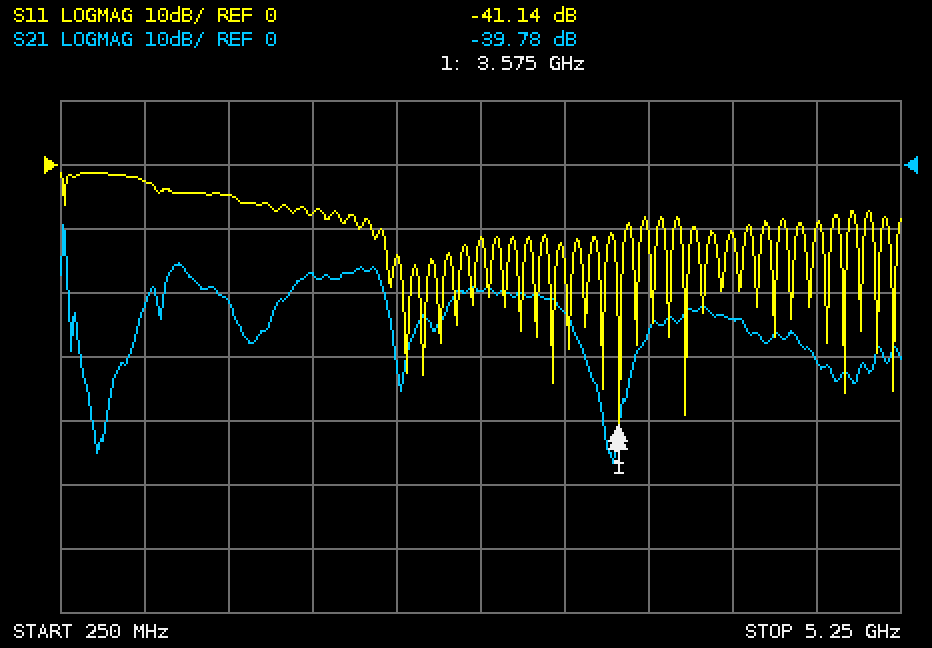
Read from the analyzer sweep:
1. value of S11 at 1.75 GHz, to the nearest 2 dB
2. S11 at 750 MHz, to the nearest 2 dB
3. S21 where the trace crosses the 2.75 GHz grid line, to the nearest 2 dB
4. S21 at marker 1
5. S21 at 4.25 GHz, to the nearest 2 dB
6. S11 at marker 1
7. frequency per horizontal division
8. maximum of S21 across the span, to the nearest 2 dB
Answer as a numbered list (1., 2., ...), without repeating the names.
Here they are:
1. -8 dB
2. -2 dB
3. -20 dB
4. -39.78 dB
5. -24 dB
6. -41.14 dB
7. 500 MHz
8. -10 dB
